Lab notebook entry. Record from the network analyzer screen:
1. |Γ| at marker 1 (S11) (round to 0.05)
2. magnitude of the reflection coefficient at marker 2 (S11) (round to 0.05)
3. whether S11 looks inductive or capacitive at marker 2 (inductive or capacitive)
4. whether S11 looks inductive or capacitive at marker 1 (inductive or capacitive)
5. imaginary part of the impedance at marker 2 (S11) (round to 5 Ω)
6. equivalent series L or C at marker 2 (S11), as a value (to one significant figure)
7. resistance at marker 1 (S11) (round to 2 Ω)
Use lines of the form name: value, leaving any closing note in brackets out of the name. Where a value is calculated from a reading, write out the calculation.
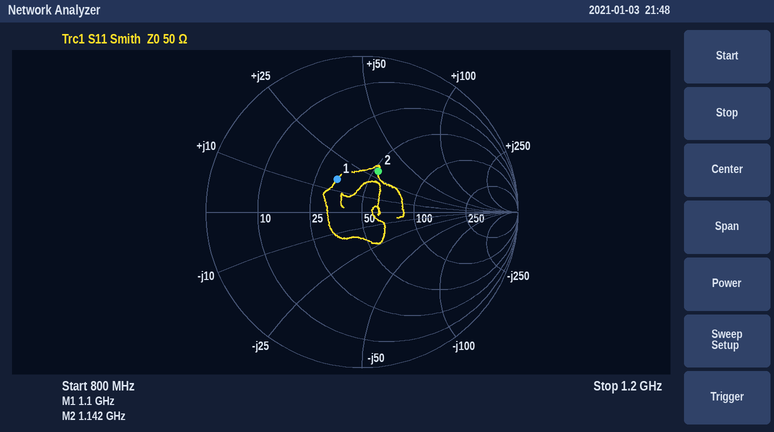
|Γ| at marker 1 (S11): 0.25
magnitude of the reflection coefficient at marker 2 (S11): 0.30
whether S11 looks inductive or capacitive at marker 2: inductive
whether S11 looks inductive or capacitive at marker 1: inductive
imaginary part of the impedance at marker 2 (S11): +30 Ω
equivalent series L or C at marker 2 (S11), as a value: L = 30 Ω/(2π × 1.142 GHz) ≈ 4 nH
resistance at marker 1 (S11): 34 Ω
